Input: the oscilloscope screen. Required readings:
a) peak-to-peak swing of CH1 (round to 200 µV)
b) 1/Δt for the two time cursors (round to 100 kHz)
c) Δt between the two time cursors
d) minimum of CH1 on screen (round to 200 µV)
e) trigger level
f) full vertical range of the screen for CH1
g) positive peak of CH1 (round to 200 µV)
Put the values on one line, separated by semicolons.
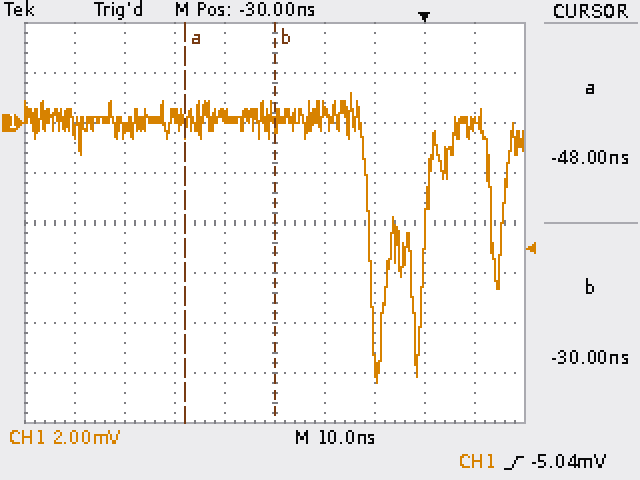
11.6 mV; 55.6 MHz; 18 ns; -10.4 mV; -5.04 mV; 16 mV; 1.2 mV
